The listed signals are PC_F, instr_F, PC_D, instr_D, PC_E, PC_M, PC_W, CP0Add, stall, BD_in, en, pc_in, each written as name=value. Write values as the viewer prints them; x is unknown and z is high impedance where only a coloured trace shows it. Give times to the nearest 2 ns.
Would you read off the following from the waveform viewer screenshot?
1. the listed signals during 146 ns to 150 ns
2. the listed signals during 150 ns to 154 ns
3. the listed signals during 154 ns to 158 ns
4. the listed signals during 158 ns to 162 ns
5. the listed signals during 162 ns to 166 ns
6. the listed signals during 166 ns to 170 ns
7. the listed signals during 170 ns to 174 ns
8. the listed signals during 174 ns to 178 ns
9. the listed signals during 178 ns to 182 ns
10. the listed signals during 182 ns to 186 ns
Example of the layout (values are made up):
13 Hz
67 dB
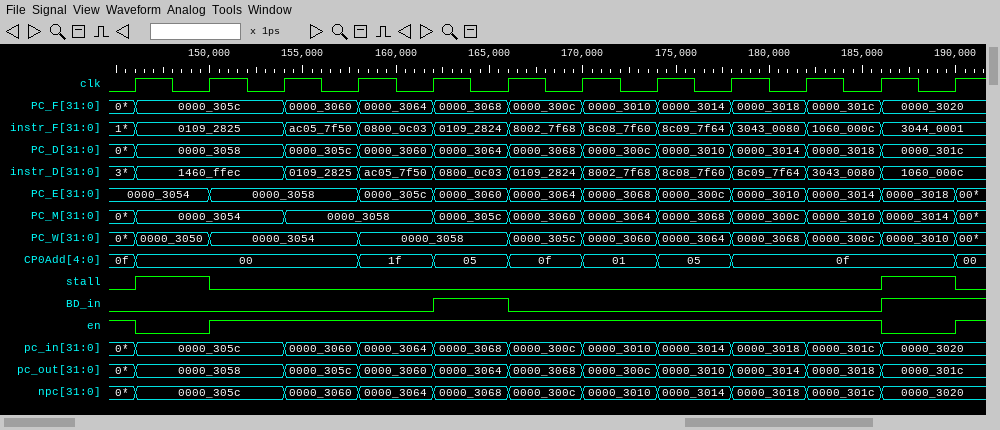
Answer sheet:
PC_F=0000_305c, instr_F=0109_2825, PC_D=0000_3058, instr_D=1460_ffec, PC_E=0000_3054, PC_M=0000_3054, PC_W=0000_3050, CP0Add=00, stall=1, BD_in=0, en=0, pc_in=0000_305c
PC_F=0000_305c, instr_F=0109_2825, PC_D=0000_3058, instr_D=1460_ffec, PC_E=0000_3058, PC_M=0000_3054, PC_W=0000_3054, CP0Add=00, stall=0, BD_in=0, en=1, pc_in=0000_305c
PC_F=0000_3060, instr_F=ac05_7f50, PC_D=0000_305c, instr_D=0109_2825, PC_E=0000_3058, PC_M=0000_3058, PC_W=0000_3054, CP0Add=00, stall=0, BD_in=0, en=1, pc_in=0000_3060
PC_F=0000_3064, instr_F=0800_0c03, PC_D=0000_3060, instr_D=ac05_7f50, PC_E=0000_305c, PC_M=0000_3058, PC_W=0000_3058, CP0Add=1f, stall=0, BD_in=0, en=1, pc_in=0000_3064
PC_F=0000_3068, instr_F=0109_2824, PC_D=0000_3064, instr_D=0800_0c03, PC_E=0000_3060, PC_M=0000_305c, PC_W=0000_3058, CP0Add=05, stall=0, BD_in=1, en=1, pc_in=0000_3068
PC_F=0000_300c, instr_F=8002_7f68, PC_D=0000_3068, instr_D=0109_2824, PC_E=0000_3064, PC_M=0000_3060, PC_W=0000_305c, CP0Add=0f, stall=0, BD_in=0, en=1, pc_in=0000_300c
PC_F=0000_3010, instr_F=8c08_7f60, PC_D=0000_300c, instr_D=8002_7f68, PC_E=0000_3068, PC_M=0000_3064, PC_W=0000_3060, CP0Add=01, stall=0, BD_in=0, en=1, pc_in=0000_3010
PC_F=0000_3014, instr_F=8c09_7f64, PC_D=0000_3010, instr_D=8c08_7f60, PC_E=0000_300c, PC_M=0000_3068, PC_W=0000_3064, CP0Add=05, stall=0, BD_in=0, en=1, pc_in=0000_3014
PC_F=0000_3018, instr_F=3043_0080, PC_D=0000_3014, instr_D=8c09_7f64, PC_E=0000_3010, PC_M=0000_300c, PC_W=0000_3068, CP0Add=0f, stall=0, BD_in=0, en=1, pc_in=0000_3018
PC_F=0000_301c, instr_F=1060_000c, PC_D=0000_3018, instr_D=3043_0080, PC_E=0000_3014, PC_M=0000_3010, PC_W=0000_300c, CP0Add=0f, stall=0, BD_in=0, en=1, pc_in=0000_301c
